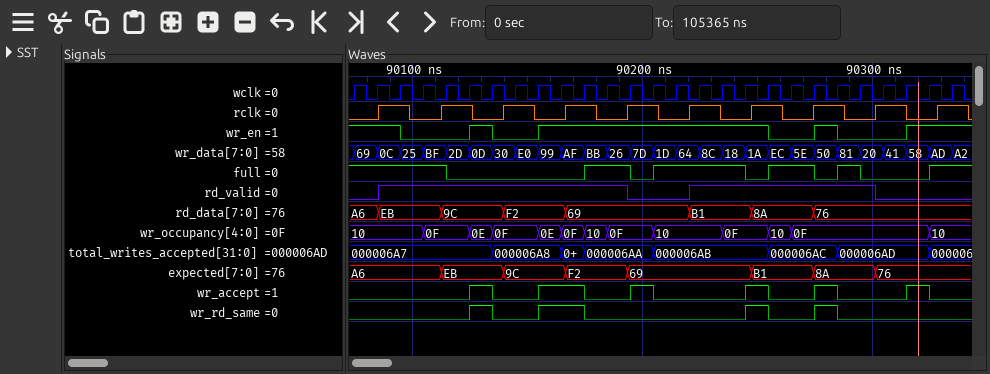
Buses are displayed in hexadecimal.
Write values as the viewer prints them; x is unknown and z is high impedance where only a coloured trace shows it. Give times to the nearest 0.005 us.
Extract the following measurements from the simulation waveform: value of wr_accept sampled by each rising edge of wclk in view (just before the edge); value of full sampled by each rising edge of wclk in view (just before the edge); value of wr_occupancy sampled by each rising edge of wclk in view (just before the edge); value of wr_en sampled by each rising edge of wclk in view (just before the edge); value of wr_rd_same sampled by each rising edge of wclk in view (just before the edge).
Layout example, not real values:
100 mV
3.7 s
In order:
0 0 0 0 0 0 1 0 0 1 1 0 0 1 0 0 0 0 1 0 0 1 0 0 0 1 0
1 1 1 1 1 0 0 0 0 0 0 1 1 0 1 1 1 1 0 1 1 0 1 0 0 0 1
10, 10, 10, 10, 0F, 0F, 0E, 0F, 0F, 0E, 0F, 10, 0F, 0F, 10, 10, 10, 0F, 0F, 10, 0F, 0F, 0F, 0F, 0F, 0F, 10
1 1 1 0 0 0 1 0 0 1 1 1 1 1 1 1 1 1 1 0 0 1 0 0 0 1 1
0 0 0 0 0 0 1 0 0 1 1 0 0 0 0 0 0 0 1 0 0 1 0 0 0 0 0
